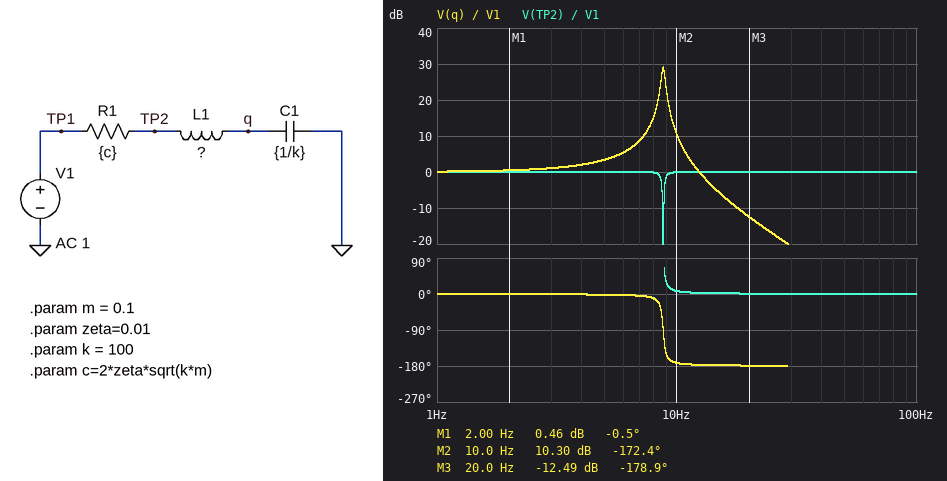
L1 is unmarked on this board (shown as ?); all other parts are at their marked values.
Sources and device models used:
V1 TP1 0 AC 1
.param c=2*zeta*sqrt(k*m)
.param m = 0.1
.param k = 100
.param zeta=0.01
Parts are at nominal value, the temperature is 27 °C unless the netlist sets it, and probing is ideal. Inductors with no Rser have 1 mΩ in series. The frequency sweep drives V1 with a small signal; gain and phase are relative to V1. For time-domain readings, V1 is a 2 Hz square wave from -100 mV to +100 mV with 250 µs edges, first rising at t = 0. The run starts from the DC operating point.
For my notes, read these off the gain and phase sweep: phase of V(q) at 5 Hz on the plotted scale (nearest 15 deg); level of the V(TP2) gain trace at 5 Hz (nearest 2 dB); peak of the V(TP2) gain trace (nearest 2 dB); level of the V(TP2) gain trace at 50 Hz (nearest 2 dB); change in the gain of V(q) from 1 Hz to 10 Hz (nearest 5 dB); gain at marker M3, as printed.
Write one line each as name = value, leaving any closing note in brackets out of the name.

phase of V(q) at 5 Hz on the plotted scale = 0 deg
level of the V(TP2) gain trace at 5 Hz = 0 dB
peak of the V(TP2) gain trace = 0 dB
level of the V(TP2) gain trace at 50 Hz = 0 dB
change in the gain of V(q) from 1 Hz to 10 Hz = 10 dB
gain at marker M3, as printed = -12.49 dB
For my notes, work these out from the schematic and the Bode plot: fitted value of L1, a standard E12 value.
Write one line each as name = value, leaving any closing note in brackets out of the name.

fitted value of L1, a standard E12 value = 33 mH
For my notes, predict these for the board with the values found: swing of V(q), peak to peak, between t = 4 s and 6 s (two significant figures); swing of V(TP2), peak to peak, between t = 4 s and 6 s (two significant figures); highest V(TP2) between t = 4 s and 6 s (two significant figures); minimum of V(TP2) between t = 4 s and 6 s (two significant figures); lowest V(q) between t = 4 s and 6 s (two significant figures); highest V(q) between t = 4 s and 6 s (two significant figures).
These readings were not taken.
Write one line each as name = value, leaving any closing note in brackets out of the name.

swing of V(q), peak to peak, between t = 4 s and 6 s = 450 mV
swing of V(TP2), peak to peak, between t = 4 s and 6 s = 210 mV
highest V(TP2) between t = 4 s and 6 s = 100 mV
minimum of V(TP2) between t = 4 s and 6 s = -100 mV
lowest V(q) between t = 4 s and 6 s = -230 mV
highest V(q) between t = 4 s and 6 s = 230 mV
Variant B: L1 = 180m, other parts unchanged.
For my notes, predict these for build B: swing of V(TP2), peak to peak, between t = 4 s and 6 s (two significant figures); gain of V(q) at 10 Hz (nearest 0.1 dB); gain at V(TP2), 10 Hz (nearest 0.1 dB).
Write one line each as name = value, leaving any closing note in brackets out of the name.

swing of V(TP2), peak to peak, between t = 4 s and 6 s = 200 mV
gain of V(q) at 10 Hz = -15.7 dB
gain at V(TP2), 10 Hz = 0 dB
